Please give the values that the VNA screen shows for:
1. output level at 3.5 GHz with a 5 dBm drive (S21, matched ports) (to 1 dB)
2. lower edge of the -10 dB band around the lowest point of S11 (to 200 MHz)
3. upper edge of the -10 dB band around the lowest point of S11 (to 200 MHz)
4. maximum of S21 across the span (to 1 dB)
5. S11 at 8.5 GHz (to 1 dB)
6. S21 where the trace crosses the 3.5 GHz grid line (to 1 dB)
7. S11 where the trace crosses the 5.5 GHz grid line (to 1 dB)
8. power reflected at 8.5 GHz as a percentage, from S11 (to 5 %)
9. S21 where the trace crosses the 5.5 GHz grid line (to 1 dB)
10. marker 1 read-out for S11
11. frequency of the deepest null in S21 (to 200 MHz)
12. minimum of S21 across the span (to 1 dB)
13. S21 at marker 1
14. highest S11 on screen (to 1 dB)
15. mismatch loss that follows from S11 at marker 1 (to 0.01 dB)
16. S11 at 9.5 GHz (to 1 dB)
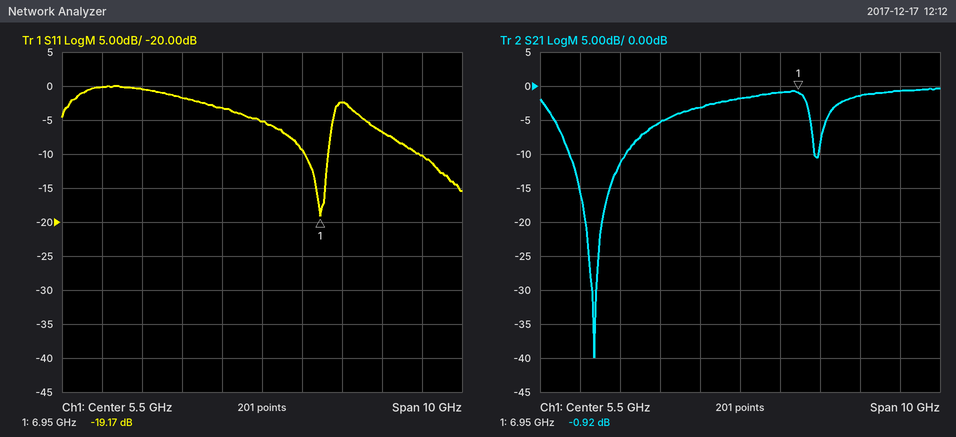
0 dBm
6.6 GHz
7.2 GHz
0 dB
-7 dB
-5 dB
-5 dB
20 %
-2 dB
-19.17 dB
1.8 GHz
-40 dB
-0.92 dB
0 dB
0.05 dB
-10 dB
